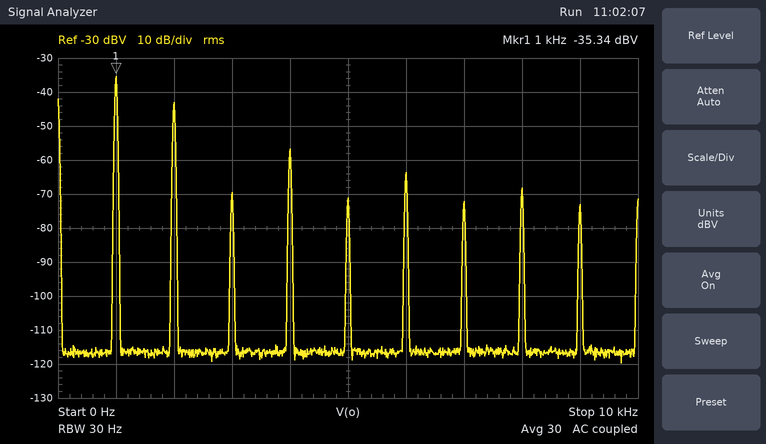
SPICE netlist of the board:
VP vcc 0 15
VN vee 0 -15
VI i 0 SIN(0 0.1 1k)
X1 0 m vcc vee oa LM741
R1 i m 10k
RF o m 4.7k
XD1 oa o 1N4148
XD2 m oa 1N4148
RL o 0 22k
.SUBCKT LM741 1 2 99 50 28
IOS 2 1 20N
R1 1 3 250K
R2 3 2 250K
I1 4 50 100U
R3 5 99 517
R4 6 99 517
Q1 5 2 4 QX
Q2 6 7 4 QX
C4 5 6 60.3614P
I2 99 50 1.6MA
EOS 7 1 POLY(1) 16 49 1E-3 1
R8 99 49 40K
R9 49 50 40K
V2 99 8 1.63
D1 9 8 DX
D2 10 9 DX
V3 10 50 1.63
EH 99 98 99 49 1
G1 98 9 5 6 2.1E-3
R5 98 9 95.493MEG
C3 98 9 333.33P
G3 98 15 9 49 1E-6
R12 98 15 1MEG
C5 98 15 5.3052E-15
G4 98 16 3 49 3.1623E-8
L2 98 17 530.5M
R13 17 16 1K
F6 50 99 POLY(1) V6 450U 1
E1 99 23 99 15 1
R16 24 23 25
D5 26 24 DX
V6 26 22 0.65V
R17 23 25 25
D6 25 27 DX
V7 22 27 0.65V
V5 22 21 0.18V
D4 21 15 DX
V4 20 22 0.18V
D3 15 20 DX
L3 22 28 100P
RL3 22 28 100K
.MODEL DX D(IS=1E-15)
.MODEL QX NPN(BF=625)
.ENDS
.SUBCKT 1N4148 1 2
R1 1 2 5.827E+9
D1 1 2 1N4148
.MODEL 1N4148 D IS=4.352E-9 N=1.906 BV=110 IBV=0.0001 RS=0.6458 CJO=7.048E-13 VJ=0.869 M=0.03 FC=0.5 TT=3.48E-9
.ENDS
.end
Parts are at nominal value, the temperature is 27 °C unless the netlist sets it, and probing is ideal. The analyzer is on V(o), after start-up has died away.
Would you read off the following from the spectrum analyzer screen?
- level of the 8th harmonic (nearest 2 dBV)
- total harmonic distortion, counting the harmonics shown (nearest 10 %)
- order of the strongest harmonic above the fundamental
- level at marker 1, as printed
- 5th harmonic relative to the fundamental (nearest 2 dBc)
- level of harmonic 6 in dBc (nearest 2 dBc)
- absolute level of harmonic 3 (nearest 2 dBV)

-68 dBV
40 %
2
-35.34 dBV
-36 dBc
-28 dBc
-70 dBV
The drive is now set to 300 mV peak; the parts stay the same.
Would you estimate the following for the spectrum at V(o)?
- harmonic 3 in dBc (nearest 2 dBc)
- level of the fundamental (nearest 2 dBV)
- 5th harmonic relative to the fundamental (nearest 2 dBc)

-42 dBc
-26 dBV
-44 dBc
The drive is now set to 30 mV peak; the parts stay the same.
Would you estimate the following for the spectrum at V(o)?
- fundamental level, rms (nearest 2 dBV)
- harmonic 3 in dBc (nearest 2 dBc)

-46 dBV
-26 dBc
